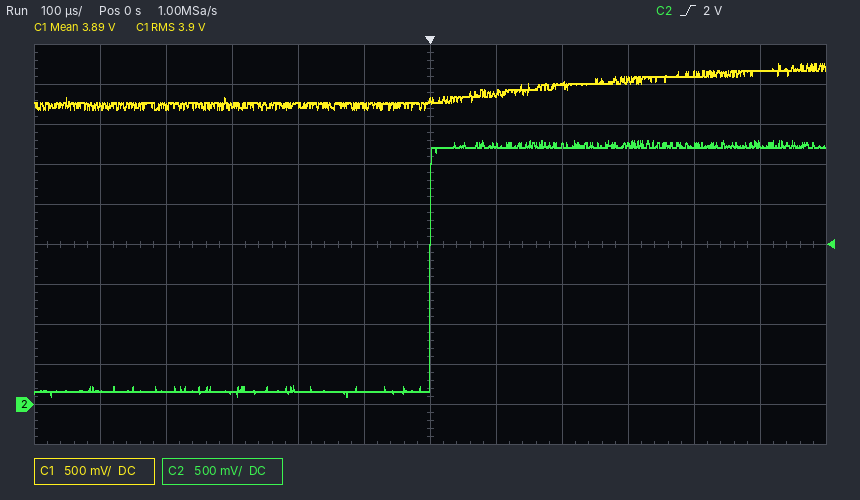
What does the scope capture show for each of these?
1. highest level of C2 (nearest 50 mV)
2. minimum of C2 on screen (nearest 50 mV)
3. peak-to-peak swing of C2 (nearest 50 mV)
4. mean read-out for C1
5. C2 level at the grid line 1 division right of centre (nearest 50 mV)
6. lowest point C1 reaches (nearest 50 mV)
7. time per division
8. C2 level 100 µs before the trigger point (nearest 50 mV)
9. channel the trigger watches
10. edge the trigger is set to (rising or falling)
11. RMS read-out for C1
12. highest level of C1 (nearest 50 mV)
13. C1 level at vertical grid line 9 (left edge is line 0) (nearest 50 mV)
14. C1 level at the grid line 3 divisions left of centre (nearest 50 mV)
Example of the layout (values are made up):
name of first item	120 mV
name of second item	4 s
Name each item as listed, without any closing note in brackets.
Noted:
highest level of C2	3.30 V
minimum of C2 on screen	100 mV
peak-to-peak swing of C2	3.20 V
mean read-out for C1	3.89 V
C2 level at the grid line 1 division right of centre	3.25 V
lowest point C1 reaches	3.70 V
time per division	100 µs
C2 level 100 µs before the trigger point	150 mV
channel the trigger watches	C2
edge the trigger is set to	rising
RMS read-out for C1	3.9 V
highest level of C1	4.25 V
C1 level at vertical grid line 9 (left edge is line 0)	4.05 V
C1 level at the grid line 3 divisions left of centre	3.75 V
